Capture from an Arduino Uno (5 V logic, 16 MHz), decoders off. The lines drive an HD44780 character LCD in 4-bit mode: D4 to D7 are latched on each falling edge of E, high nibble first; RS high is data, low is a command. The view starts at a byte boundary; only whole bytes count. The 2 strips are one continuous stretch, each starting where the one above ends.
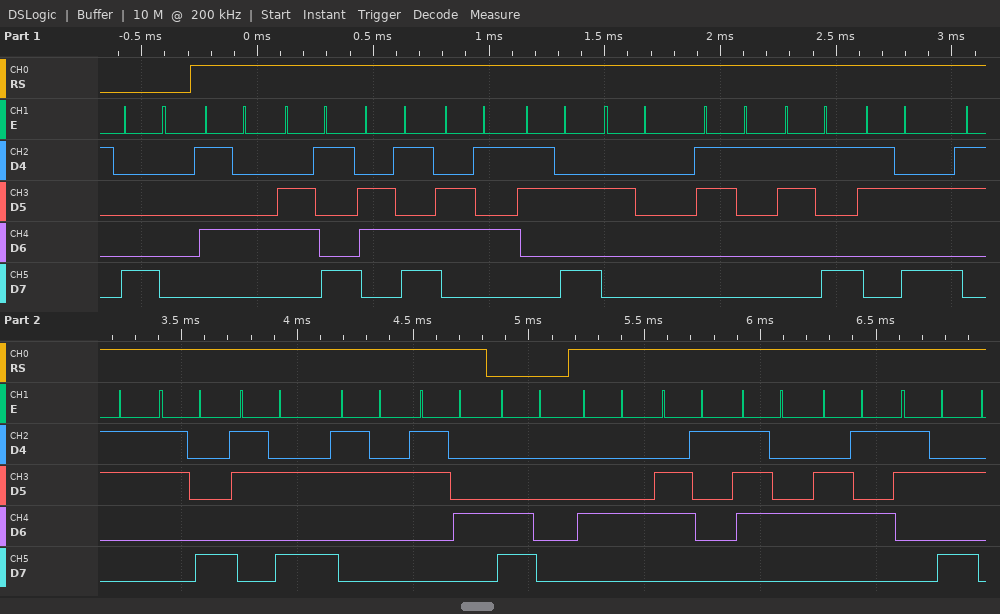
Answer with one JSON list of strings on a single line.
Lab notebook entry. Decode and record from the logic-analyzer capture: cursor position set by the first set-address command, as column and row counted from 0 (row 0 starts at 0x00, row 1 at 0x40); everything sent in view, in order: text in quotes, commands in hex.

["column 0, row 0", "0x80 \"Time: 19:38:24\" 0xC0 \"Date:\""]
